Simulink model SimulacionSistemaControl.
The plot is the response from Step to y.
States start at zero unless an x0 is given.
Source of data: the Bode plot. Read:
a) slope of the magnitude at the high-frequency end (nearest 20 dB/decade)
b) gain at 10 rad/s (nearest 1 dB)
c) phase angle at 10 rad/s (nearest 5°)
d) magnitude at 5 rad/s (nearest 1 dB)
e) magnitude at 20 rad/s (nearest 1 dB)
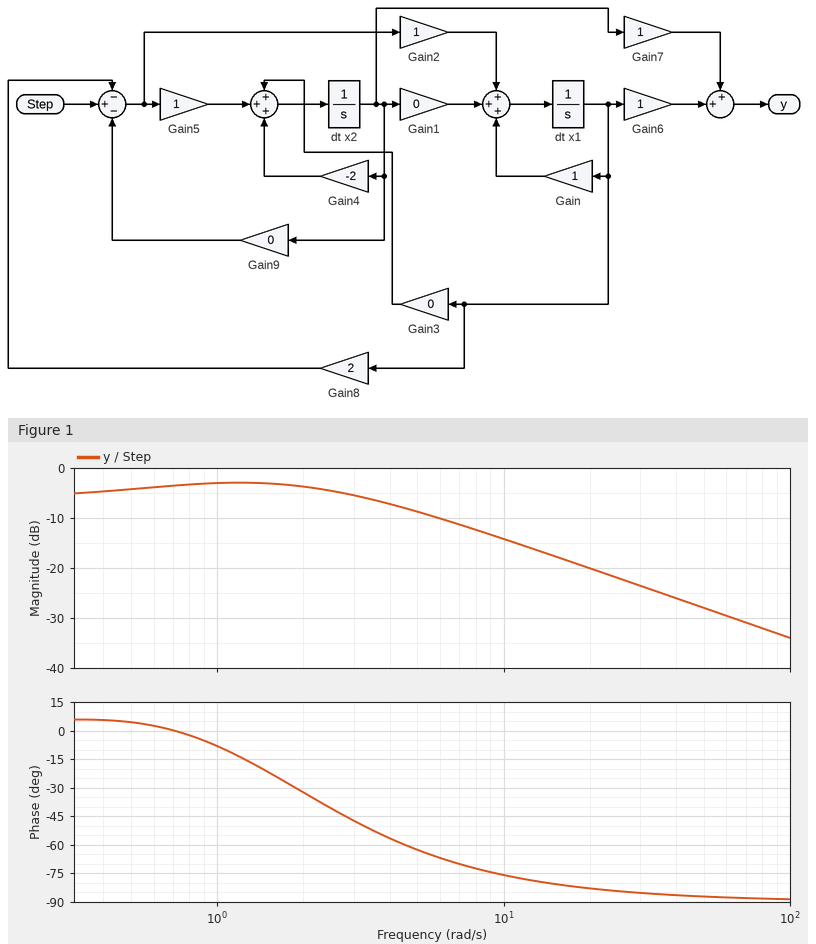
-20 dB/decade
-14 dB
-75°
-9 dB
-20 dB
